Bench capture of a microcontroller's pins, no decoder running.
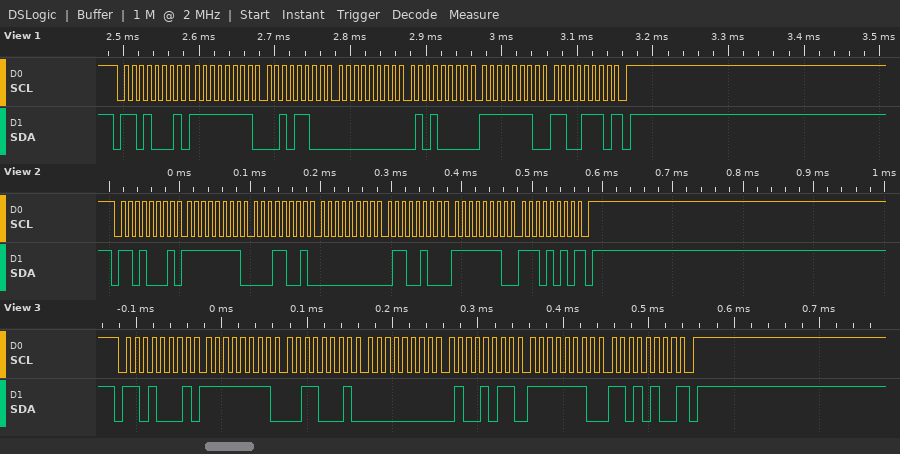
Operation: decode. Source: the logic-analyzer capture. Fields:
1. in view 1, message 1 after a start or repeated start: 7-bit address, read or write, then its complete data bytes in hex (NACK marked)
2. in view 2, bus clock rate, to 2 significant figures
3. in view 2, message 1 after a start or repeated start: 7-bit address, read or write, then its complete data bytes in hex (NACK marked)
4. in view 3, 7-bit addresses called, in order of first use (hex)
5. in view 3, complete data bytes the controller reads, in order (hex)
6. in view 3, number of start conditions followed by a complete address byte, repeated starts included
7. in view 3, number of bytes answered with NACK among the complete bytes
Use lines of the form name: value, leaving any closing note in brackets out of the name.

in view 1, message 1 after a start or repeated start: 7-bit address, read or write, then its complete data bytes in hex: 0x68 read: FF 2C 00 50 FE CE NACK
in view 2, bus clock rate, to 2 significant figures: 100 kHz
in view 2, message 1 after a start or repeated start: 7-bit address, read or write, then its complete data bytes in hex: 0x68 read: FF 19 00 64 FE EA NACK
in view 3, 7-bit addresses called, in order of first use: 0x68
in view 3, complete data bytes the controller reads, in order: FF 31 00 4B FE D4
in view 3, number of start conditions followed by a complete address byte, repeated starts included: 1
in view 3, number of bytes answered with NACK among the complete bytes: 1
